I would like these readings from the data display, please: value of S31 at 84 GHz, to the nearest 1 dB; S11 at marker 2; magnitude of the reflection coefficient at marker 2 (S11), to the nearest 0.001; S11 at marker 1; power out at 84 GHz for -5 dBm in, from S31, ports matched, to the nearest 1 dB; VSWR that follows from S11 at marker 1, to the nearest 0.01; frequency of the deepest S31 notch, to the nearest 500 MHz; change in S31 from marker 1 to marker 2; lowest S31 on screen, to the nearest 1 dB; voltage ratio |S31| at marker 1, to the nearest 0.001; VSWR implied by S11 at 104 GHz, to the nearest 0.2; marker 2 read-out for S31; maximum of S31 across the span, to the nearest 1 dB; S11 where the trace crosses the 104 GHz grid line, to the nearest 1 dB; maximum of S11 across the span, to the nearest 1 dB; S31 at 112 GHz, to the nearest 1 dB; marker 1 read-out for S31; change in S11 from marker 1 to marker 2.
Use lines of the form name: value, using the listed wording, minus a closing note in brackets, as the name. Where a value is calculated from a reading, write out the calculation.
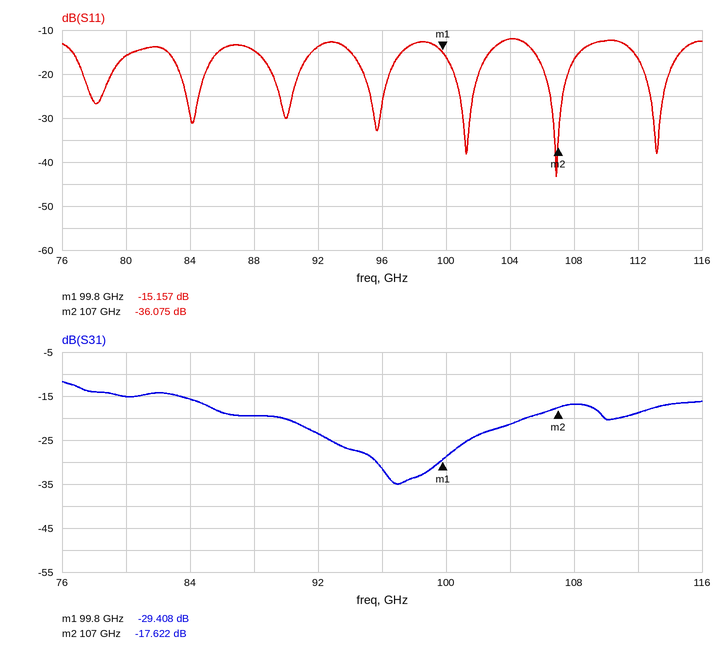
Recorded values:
value of S31 at 84 GHz, to the nearest 1 dB: -16 dB
S11 at marker 2: -36.075 dB
magnitude of the reflection coefficient at marker 2 (S11), to the nearest 0.001: 10^(-36.075/20) ≈ 0.016
S11 at marker 1: -15.157 dB
power out at 84 GHz for -5 dBm in, from S31, ports matched, to the nearest 1 dB: -5 dBm + (-16 dB) = -21 dBm
VSWR that follows from S11 at marker 1, to the nearest 0.01: (1 + 0.1746)/(1 − 0.1746) ≈ 1.42
frequency of the deepest S31 notch, to the nearest 500 MHz: 97.0 GHz
change in S31 from marker 1 to marker 2: -17.622 − (-29.408) = 11.786 dB
lowest S31 on screen, to the nearest 1 dB: -35 dB
voltage ratio |S31| at marker 1, to the nearest 0.001: 10^(-29.408/20) ≈ 0.034
VSWR implied by S11 at 104 GHz, to the nearest 0.2: |Γ| = 10^(-12/20) = 0.2512; VSWR = (1 + 0.2512)/(1 − 0.2512) ≈ 1.67, so 1.6 to the nearest 0.2
marker 2 read-out for S31: -17.622 dB
maximum of S31 across the span, to the nearest 1 dB: -12 dB
S11 where the trace crosses the 104 GHz grid line, to the nearest 1 dB: -12 dB
maximum of S11 across the span, to the nearest 1 dB: -12 dB
S31 at 112 GHz, to the nearest 1 dB: -19 dB
marker 1 read-out for S31: -29.408 dB
change in S11 from marker 1 to marker 2: -36.075 − (-15.157) = -20.918 dB
